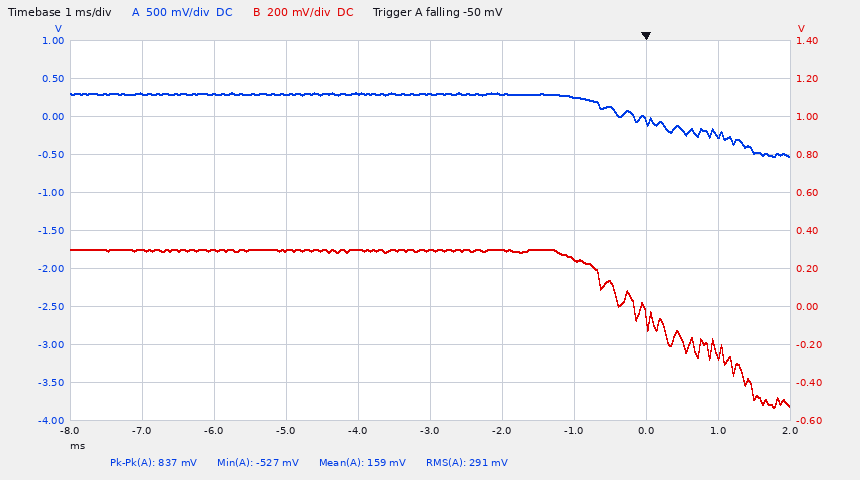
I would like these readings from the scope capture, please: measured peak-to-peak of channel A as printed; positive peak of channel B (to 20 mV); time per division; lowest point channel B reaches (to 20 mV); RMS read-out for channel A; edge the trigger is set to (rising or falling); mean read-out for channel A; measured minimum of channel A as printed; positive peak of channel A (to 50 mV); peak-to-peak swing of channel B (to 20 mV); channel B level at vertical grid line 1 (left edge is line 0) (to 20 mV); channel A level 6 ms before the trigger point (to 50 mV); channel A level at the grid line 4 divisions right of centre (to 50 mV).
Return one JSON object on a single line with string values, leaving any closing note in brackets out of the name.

{"measured peak-to-peak of channel A as printed": "837 mV", "positive peak of channel B": "300 mV", "time per division": "1 ms", "lowest point channel B reaches": "-540 mV", "RMS read-out for channel A": "291 mV", "edge the trigger is set to": "falling", "mean read-out for channel A": "159 mV", "measured minimum of channel A as printed": "-527 mV", "positive peak of channel A": "300 mV", "peak-to-peak swing of channel B": "840 mV", "channel B level at vertical grid line 1 (left edge is line 0)": "300 mV", "channel A level 6 ms before the trigger point": "300 mV", "channel A level at the grid line 4 divisions right of centre": "-250 mV"}
